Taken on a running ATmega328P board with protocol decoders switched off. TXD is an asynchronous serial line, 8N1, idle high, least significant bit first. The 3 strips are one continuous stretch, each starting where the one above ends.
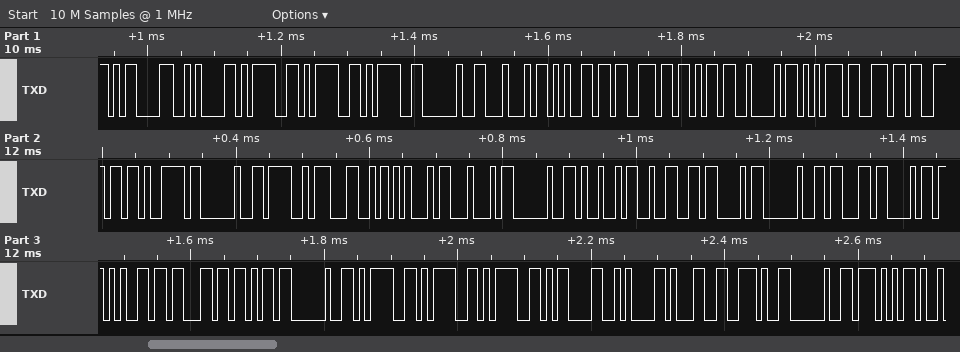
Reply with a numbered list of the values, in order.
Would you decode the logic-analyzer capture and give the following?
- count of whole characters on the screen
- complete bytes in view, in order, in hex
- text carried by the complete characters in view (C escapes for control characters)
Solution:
1. 40
2. 0D 0A 3D 3D 3D 20 44 65 73 6B 42 75 6E 6E 79 20 4F 4C 45 44 20 49 32 43 20 63 68 65 63 6B 20 3D 3D 3D 0D 0A 31 2E 20 57
3. "\r\n=== DeskBunny OLED I2C check ===\r\n1. W"
